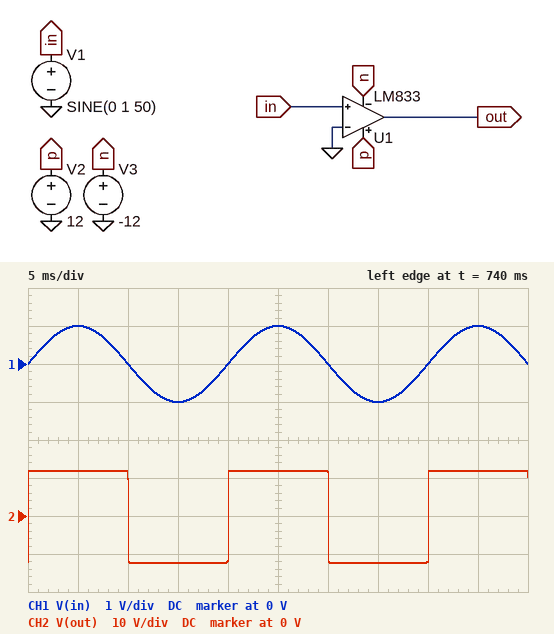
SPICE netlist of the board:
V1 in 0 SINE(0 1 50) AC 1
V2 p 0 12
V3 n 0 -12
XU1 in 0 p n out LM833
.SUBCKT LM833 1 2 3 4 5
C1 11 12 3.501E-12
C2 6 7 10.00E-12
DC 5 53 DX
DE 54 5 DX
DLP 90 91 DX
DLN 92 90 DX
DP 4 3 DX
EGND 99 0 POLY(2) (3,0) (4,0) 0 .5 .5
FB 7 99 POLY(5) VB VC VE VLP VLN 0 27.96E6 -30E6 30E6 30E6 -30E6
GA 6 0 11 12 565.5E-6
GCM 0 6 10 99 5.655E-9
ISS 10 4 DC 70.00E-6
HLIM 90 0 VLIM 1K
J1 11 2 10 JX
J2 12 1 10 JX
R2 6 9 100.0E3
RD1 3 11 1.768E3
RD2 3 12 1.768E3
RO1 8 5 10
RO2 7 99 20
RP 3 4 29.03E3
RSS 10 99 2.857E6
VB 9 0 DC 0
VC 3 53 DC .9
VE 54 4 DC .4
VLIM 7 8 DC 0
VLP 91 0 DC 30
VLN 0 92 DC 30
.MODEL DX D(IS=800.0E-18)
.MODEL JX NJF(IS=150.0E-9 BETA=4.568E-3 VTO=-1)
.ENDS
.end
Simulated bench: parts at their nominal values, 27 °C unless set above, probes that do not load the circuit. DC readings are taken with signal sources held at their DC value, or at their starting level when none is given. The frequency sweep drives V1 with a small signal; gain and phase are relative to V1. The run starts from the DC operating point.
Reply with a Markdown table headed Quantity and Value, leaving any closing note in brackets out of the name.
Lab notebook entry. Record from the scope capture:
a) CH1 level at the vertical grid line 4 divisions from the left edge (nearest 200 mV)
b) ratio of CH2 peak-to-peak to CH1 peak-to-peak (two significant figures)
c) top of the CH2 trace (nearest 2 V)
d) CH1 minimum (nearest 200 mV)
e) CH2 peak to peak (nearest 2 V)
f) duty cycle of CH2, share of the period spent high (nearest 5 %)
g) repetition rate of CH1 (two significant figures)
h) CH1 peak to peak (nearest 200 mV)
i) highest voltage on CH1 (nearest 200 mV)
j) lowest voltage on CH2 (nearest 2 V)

| Quantity | Value |
|---|---|
| CH1 level at the vertical grid line 4 divisions from the left edge | 0 V |
| ratio of CH2 peak-to-peak to CH1 peak-to-peak | 12 |
| top of the CH2 trace | 12 V |
| CH1 minimum | -1.0 V |
| CH2 peak to peak | 24 V |
| duty cycle of CH2, share of the period spent high | 50 % |
| repetition rate of CH1 | 50 Hz |
| CH1 peak to peak | 2.0 V |
| highest voltage on CH1 | 1.0 V |
| lowest voltage on CH2 | -12 V |
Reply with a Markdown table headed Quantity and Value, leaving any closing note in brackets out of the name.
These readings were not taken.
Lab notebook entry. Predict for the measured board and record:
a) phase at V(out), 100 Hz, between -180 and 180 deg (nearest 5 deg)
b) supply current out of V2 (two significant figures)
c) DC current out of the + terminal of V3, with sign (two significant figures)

| Quantity | Value |
|---|---|
| phase at V(out), 100 Hz, between -180 and 180 deg | -75 deg |
| supply current out of V2 | 900 µA |
| DC current out of the + terminal of V3, with sign | -900 µA |
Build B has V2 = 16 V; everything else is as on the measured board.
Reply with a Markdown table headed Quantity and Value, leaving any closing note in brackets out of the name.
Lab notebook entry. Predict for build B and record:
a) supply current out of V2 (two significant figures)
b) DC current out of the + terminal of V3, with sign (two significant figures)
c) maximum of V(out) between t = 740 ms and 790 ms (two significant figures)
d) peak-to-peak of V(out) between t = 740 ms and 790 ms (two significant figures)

| Quantity | Value |
|---|---|
| supply current out of V2 | 1.0 mA |
| DC current out of the + terminal of V3, with sign | -1.0 mA |
| maximum of V(out) between t = 740 ms and 790 ms | 16 V |
| peak-to-peak of V(out) between t = 740 ms and 790 ms | 28 V |
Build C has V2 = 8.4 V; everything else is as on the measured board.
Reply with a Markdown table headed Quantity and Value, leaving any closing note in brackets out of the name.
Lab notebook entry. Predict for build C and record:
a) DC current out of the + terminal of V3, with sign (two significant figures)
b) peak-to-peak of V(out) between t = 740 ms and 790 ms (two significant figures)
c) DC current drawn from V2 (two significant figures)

| Quantity | Value |
|---|---|
| DC current out of the + terminal of V3, with sign | -770 µA |
| peak-to-peak of V(out) between t = 740 ms and 790 ms | 20 V |
| DC current drawn from V2 | 770 µA |
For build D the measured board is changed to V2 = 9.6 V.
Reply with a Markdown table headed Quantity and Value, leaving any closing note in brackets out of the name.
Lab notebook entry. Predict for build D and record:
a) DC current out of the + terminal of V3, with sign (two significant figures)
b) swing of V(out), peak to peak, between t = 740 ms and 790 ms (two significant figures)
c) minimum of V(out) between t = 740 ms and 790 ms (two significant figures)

| Quantity | Value |
|---|---|
| DC current out of the + terminal of V3, with sign | -810 µA |
| swing of V(out), peak to peak, between t = 740 ms and 790 ms | 22 V |
| minimum of V(out) between t = 740 ms and 790 ms | -12 V |
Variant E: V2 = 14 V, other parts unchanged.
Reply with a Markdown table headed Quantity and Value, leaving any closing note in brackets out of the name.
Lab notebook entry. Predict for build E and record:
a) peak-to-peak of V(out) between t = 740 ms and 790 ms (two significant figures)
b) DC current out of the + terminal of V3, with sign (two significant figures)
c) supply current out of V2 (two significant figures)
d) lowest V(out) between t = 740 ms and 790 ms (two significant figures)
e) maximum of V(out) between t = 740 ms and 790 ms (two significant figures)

| Quantity | Value |
|---|---|
| peak-to-peak of V(out) between t = 740 ms and 790 ms | 26 V |
| DC current out of the + terminal of V3, with sign | -970 µA |
| supply current out of V2 | 970 µA |
| lowest V(out) between t = 740 ms and 790 ms | -12 V |
| maximum of V(out) between t = 740 ms and 790 ms | 14 V |
